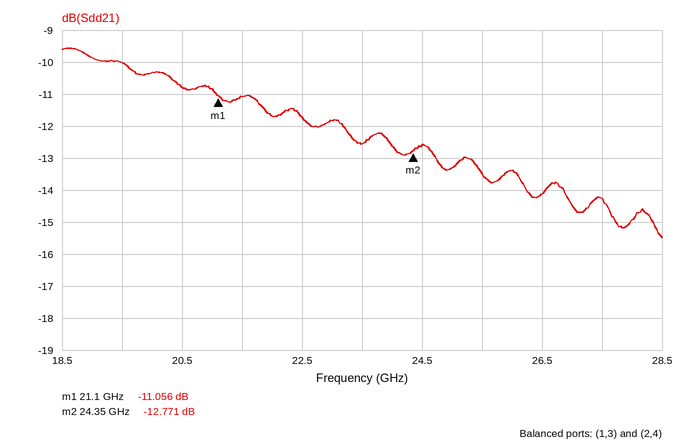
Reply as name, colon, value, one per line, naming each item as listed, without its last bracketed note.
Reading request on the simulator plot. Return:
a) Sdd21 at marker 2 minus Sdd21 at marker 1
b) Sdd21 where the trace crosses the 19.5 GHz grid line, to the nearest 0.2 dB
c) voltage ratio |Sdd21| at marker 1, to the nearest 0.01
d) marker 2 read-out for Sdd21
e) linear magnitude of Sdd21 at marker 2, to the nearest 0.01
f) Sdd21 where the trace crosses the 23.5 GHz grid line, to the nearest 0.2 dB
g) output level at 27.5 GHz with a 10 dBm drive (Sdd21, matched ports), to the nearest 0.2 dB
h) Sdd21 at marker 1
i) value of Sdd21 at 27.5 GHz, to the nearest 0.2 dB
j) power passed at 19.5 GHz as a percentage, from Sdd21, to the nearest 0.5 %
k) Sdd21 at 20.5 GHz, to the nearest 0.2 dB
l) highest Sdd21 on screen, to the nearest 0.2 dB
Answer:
Sdd21 at marker 2 minus Sdd21 at marker 1: -1.715 dB
Sdd21 where the trace crosses the 19.5 GHz grid line, to the nearest 0.2 dB: -10.0 dB
voltage ratio |Sdd21| at marker 1, to the nearest 0.01: 0.28
marker 2 read-out for Sdd21: -12.771 dB
linear magnitude of Sdd21 at marker 2, to the nearest 0.01: 0.23
Sdd21 where the trace crosses the 23.5 GHz grid line, to the nearest 0.2 dB: -12.6 dB
output level at 27.5 GHz with a 10 dBm drive (Sdd21, matched ports), to the nearest 0.2 dB: -4.2 dBm
Sdd21 at marker 1: -11.056 dB
value of Sdd21 at 27.5 GHz, to the nearest 0.2 dB: -14.2 dB
power passed at 19.5 GHz as a percentage, from Sdd21, to the nearest 0.5 %: 10.0 %
Sdd21 at 20.5 GHz, to the nearest 0.2 dB: -10.8 dB
highest Sdd21 on screen, to the nearest 0.2 dB: -9.6 dB
